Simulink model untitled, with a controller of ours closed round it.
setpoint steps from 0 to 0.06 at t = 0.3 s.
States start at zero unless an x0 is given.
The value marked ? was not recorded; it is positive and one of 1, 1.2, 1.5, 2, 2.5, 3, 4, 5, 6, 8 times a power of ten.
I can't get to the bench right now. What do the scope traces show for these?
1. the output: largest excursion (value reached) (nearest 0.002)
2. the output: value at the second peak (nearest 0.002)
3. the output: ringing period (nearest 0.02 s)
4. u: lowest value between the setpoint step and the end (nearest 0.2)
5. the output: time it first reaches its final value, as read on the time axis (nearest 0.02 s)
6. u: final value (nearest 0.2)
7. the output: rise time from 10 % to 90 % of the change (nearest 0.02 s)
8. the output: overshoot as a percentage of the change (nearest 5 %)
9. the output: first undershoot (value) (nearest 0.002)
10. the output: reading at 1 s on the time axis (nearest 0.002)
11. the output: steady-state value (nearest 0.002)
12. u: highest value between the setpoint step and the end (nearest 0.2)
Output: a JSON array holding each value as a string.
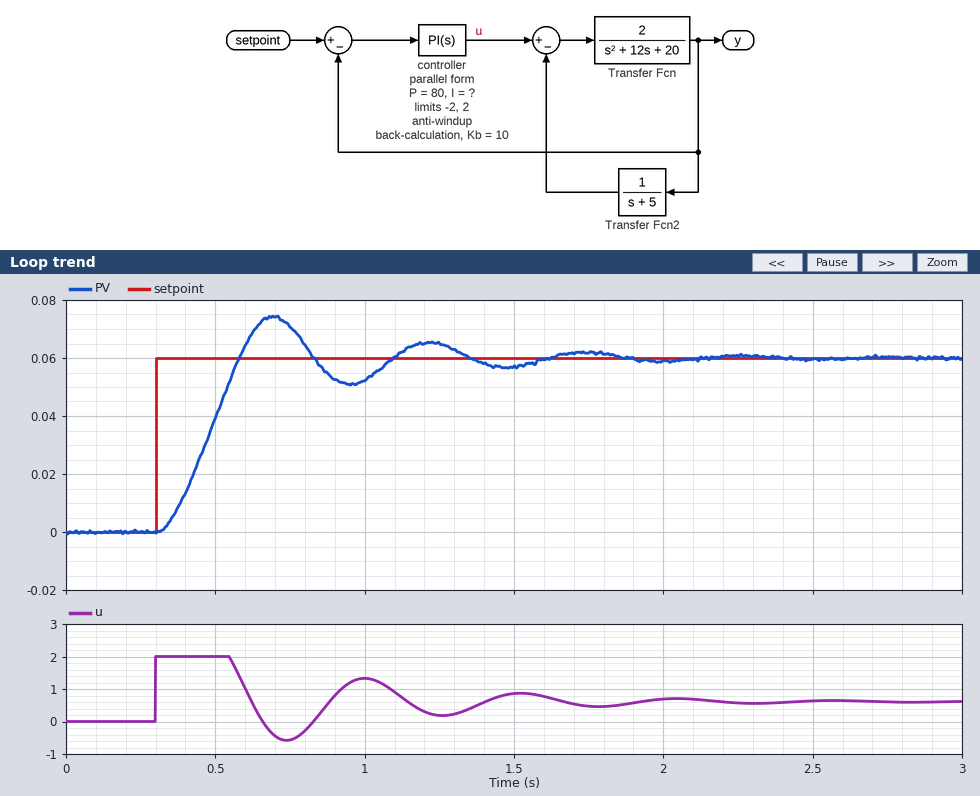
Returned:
["0.074", "0.066", "0.52 s", "-0.6", "0.58 s", "0.6", "0.20 s", "25 %", "0.050", "0.052", "0.060", "2.0"]
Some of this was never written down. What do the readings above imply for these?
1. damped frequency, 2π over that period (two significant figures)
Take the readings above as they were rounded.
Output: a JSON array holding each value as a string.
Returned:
["12 rad/s"]
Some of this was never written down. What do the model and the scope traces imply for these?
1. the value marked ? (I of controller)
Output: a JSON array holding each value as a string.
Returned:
["600"]
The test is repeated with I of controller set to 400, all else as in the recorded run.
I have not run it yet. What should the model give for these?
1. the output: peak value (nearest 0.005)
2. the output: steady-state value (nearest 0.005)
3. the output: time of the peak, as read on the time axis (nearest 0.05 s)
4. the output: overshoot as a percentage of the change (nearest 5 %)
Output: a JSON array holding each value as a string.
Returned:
["0.070", "0.060", "0.70 s", "15 %"]
